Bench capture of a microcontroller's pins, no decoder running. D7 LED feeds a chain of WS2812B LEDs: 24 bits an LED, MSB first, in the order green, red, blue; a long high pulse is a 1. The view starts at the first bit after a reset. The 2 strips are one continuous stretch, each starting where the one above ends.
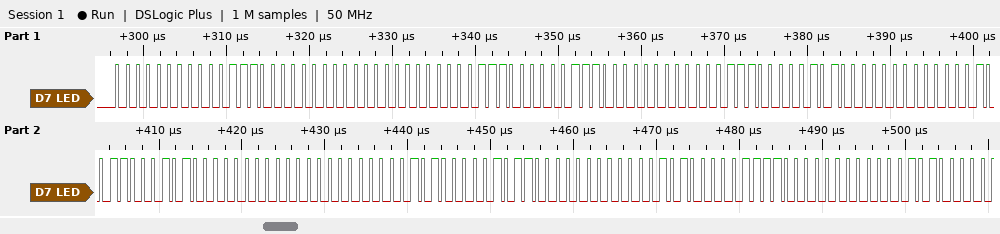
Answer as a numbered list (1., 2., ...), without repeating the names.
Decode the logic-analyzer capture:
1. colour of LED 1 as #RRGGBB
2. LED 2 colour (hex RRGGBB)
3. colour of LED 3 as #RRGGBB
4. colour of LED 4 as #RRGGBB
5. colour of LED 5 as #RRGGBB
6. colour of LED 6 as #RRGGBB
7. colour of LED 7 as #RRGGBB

1. #1C0000
2. #1C000E
3. #1C0014
4. #130014
5. #000014
6. #001614
7. #001E14
